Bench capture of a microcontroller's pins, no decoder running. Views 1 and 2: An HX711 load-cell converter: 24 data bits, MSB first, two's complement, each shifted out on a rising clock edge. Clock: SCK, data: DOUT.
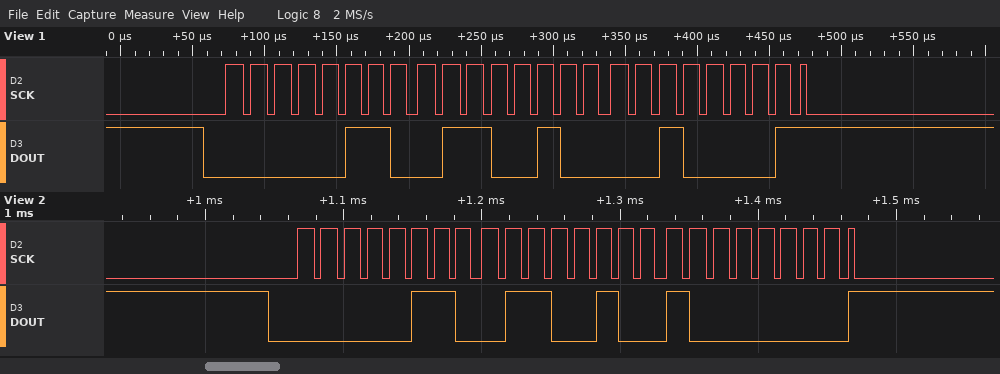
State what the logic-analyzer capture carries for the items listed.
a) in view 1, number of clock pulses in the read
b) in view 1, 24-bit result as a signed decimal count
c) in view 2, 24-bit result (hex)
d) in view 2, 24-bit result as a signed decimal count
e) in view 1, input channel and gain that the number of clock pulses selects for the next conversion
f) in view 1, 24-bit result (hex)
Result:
25
418849
0x066480
418944
channel A, gain 128
0x066421
